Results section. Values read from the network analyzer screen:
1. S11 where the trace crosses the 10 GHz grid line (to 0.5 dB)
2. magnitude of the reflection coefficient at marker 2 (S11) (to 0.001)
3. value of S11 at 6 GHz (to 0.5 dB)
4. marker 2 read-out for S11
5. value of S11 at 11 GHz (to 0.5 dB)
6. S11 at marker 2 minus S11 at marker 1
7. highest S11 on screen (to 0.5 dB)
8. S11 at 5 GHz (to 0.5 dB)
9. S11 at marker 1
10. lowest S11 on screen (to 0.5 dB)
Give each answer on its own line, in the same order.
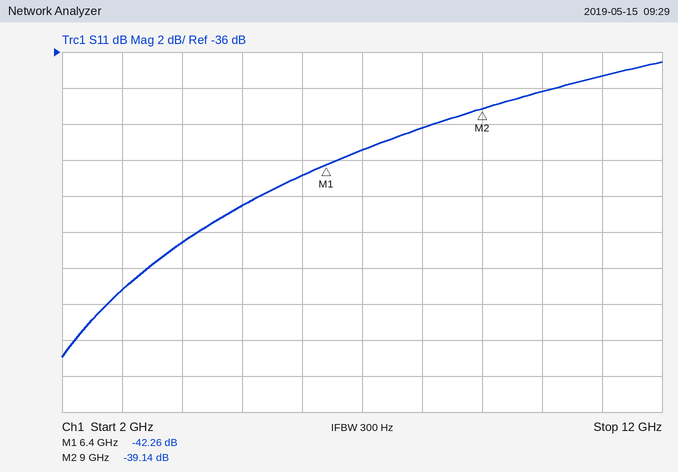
-38.0 dB
0.011
-43.0 dB
-39.14 dB
-37.5 dB
3.12 dB
-36.5 dB
-44.5 dB
-42.26 dB
-53.0 dB
